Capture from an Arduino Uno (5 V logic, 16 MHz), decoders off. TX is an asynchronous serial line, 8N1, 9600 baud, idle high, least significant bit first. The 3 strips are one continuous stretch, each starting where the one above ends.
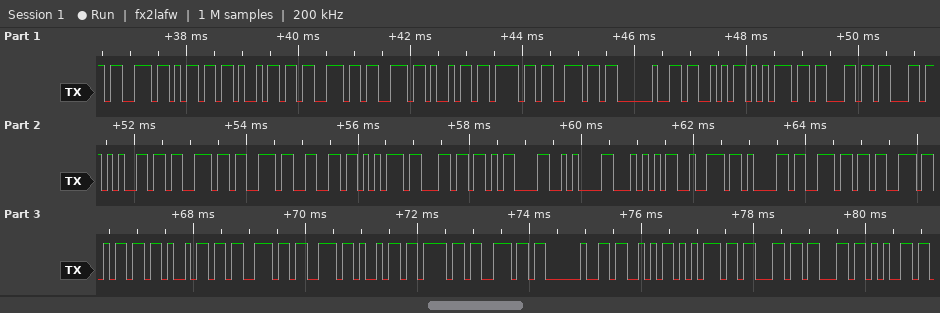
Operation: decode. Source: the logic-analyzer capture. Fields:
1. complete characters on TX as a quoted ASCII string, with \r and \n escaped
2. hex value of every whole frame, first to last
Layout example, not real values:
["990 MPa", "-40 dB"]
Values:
["\"smission Successful\\r\\nTransmission Succe\"", "73 6D 69 73 73 69 6F 6E 20 53 75 63 63 65 73 73 66 75 6C 0D 0A 54 72 61 6E 73 6D 69 73 73 69 6F 6E 20 53 75 63 63 65"]
